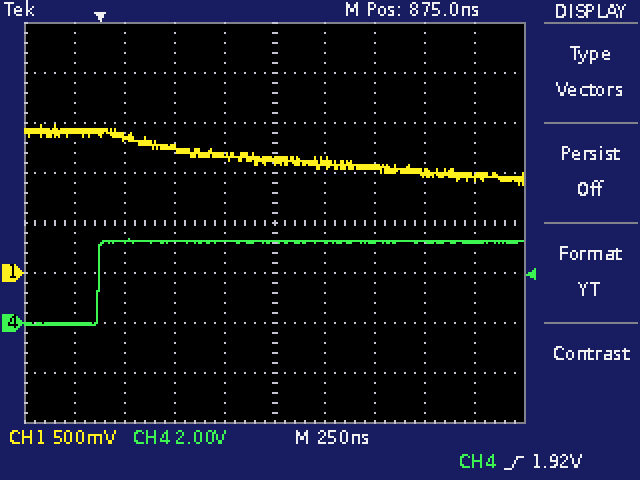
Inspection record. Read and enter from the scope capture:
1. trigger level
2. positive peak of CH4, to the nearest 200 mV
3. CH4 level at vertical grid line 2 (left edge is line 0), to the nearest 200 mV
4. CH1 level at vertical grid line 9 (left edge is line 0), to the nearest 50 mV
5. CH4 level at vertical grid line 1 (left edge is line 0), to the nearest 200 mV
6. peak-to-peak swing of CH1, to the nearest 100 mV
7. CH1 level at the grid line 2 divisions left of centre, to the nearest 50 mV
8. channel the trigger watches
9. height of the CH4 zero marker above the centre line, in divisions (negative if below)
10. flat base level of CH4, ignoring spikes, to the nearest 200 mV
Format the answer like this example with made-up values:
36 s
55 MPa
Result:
1.92 V
3.4 V
3.2 V
950 mV
0.0 V
600 mV
1.25 V
CH4
-2.0 div
0.0 V
